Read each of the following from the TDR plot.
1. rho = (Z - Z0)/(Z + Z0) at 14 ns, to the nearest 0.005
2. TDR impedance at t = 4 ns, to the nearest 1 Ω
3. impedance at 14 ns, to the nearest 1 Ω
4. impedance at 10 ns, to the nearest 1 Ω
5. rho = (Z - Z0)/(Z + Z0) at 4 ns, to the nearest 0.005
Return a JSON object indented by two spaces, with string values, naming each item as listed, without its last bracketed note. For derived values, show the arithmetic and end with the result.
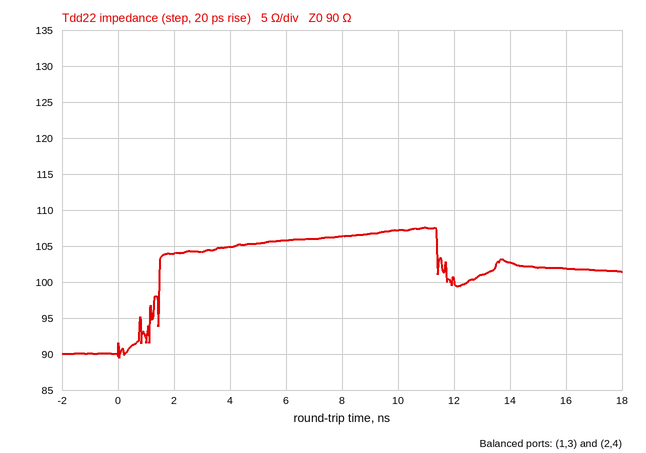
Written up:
{
  "rho = (Z - Z0)/(Z + Z0) at 14 ns, to the nearest 0.005": "(103 − 90)/(103 + 90) ≈ +0.0674, so +0.065 to the nearest 0.005",
  "TDR impedance at t = 4 ns, to the nearest 1 Ω": "105 Ω",
  "impedance at 14 ns, to the nearest 1 Ω": "103 Ω",
  "impedance at 10 ns, to the nearest 1 Ω": "107 Ω",
  "rho = (Z - Z0)/(Z + Z0) at 4 ns, to the nearest 0.005": "(105 − 90)/(105 + 90) ≈ +0.0769, so +0.075 to the nearest 0.005"
}
